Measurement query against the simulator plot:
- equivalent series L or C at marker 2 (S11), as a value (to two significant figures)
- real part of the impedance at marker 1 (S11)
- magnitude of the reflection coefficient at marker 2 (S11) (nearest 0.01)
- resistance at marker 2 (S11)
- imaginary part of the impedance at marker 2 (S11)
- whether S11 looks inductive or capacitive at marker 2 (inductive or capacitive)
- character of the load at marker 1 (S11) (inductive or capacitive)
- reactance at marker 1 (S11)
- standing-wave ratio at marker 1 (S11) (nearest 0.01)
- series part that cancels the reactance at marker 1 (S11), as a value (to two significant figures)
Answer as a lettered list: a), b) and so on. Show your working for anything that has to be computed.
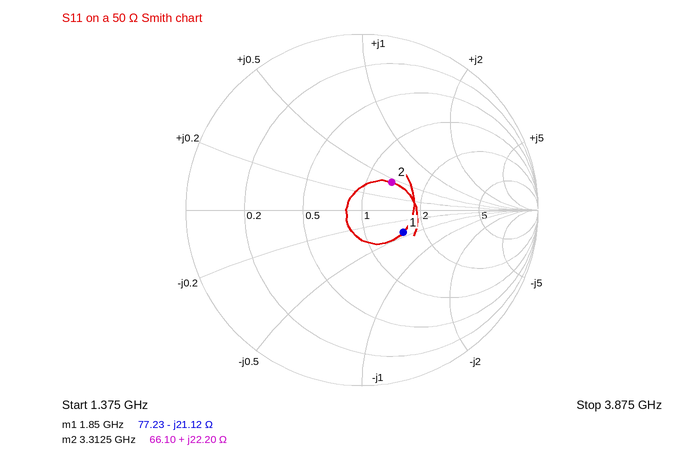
a) L = 22.2 Ω/(2π × 3.3125 GHz) ≈ 1.1 nH
b) 77.23 Ω
c) 0.23
d) 66.10 Ω
e) +22.20 Ω
f) inductive
g) capacitive
h) -21.12 Ω
i) 1.73
j) L = 21.12 Ω/(2π × 1.85 GHz) ≈ 1.8 nH
